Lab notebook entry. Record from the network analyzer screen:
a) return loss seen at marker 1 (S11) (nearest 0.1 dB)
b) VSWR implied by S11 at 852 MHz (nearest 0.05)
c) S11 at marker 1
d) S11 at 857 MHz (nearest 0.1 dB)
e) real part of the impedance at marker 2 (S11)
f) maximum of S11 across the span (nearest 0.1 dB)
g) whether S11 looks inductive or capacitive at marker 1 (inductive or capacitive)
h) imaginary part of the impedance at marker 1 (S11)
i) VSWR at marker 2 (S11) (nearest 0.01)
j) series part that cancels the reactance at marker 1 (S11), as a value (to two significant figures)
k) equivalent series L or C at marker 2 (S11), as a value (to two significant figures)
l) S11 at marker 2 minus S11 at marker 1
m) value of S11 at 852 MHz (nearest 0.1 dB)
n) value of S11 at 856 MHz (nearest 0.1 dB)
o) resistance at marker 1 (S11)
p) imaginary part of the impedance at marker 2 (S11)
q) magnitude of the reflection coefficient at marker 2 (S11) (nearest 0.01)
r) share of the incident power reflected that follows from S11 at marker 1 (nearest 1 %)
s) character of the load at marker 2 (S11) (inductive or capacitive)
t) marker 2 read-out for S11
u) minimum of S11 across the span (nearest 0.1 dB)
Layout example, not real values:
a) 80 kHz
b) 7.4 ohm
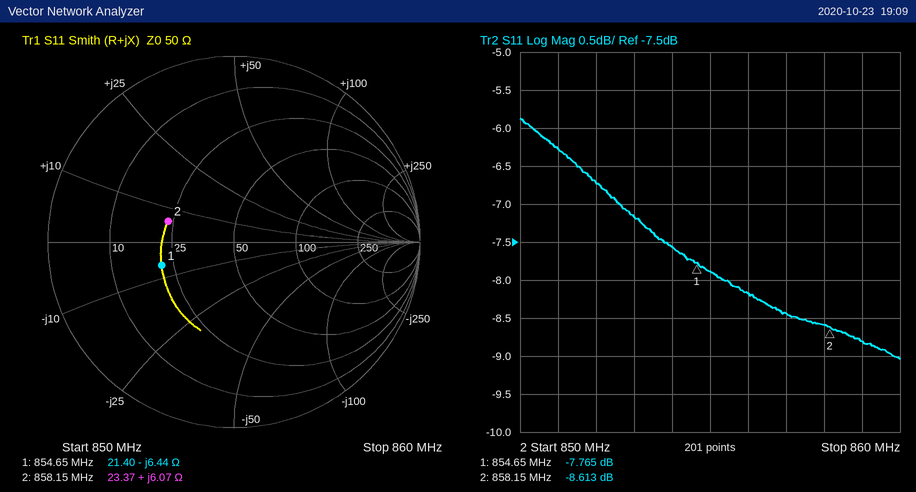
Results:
a) 7.8 dB
b) 2.70
c) -7.765 dB
d) -8.4 dB
e) 23.37 Ω
f) -5.9 dB
g) capacitive
h) -6.44 Ω
i) 2.18
j) 1.2 nH
k) 1.1 nH
l) -0.848 dB
m) -6.7 dB
n) -8.2 dB
o) 21.40 Ω
p) +6.07 Ω
q) 0.37
r) 17 %
s) inductive
t) -8.613 dB
u) -9.0 dB
